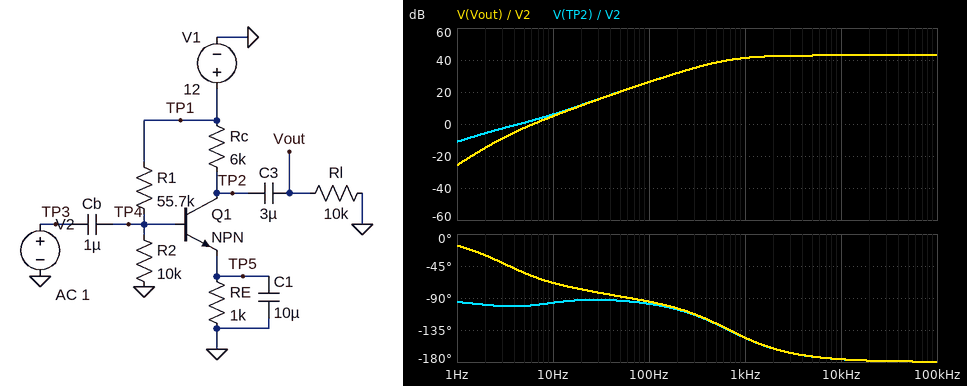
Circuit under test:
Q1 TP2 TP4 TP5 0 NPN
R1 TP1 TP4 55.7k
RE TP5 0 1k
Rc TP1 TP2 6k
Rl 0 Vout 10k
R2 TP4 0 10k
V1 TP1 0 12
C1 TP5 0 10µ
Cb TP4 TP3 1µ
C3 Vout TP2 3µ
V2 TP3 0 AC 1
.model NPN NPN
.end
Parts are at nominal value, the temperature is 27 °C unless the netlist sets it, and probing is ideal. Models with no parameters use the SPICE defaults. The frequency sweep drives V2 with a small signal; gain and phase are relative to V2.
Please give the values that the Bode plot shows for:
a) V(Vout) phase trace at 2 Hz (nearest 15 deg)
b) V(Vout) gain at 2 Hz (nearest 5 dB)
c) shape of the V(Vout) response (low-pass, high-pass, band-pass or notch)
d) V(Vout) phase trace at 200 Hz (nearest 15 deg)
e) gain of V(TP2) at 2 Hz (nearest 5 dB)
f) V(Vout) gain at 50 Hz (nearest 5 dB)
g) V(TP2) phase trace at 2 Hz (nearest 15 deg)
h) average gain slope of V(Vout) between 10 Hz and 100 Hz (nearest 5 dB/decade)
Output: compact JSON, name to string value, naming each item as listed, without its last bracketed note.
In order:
{"V(Vout) phase trace at 2 Hz": "-30 deg", "V(Vout) gain at 2 Hz": "-15 dB", "shape of the V(Vout) response": "high-pass", "V(Vout) phase trace at 200 Hz": "-105 deg", "gain of V(TP2) at 2 Hz": "-5 dB", "V(Vout) gain at 50 Hz": "20 dB", "V(TP2) phase trace at 2 Hz": "-105 deg", "average gain slope of V(Vout) between 10 Hz and 100 Hz": "20 dB/decade"}
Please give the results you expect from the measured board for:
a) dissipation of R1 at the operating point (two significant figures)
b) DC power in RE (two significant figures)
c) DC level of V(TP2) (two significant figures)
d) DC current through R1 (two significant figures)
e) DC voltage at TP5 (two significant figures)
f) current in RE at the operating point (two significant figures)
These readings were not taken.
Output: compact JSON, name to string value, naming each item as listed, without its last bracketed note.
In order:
{"dissipation of R1 at the operating point": "1.9 mW", "DC power in RE": "940 µW", "DC level of V(TP2)": "6.2 V", "DC current through R1": "180 µA", "DC voltage at TP5": "970 mV", "current in RE at the operating point": "970 µA"}
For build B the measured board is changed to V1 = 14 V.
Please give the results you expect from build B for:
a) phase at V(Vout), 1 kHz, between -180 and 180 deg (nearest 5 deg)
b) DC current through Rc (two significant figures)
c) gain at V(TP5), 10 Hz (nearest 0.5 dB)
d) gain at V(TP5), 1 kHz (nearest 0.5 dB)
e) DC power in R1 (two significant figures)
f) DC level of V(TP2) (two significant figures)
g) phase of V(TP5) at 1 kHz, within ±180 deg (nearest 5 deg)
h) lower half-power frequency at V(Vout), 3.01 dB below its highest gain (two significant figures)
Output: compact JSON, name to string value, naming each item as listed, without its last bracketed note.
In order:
{"phase at V(Vout), 1 kHz, between -180 and 180 deg": "-140 deg", "DC current through Rc": "1.2 mA", "gain at V(TP5), 10 Hz": "-7.5 dB", "gain at V(TP5), 1 kHz": "-4.5 dB", "DC power in R1": "2.6 mW", "DC level of V(TP2)": "6.6 V", "phase of V(TP5) at 1 kHz, within ±180 deg": "-50 deg", "lower half-power frequency at V(Vout), 3.01 dB below its highest gain": "860 Hz"}
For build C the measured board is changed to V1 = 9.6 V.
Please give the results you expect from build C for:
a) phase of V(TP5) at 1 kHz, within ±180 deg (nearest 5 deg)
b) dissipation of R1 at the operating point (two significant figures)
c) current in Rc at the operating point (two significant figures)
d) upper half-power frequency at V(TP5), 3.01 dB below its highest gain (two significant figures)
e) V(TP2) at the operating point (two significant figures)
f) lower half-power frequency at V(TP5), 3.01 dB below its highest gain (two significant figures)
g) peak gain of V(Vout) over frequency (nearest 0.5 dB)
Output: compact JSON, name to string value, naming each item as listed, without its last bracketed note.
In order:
{"phase of V(TP5) at 1 kHz, within ±180 deg": "-65 deg", "dissipation of R1 at the operating point": "1.2 mW", "current in Rc at the operating point": "640 µA", "upper half-power frequency at V(TP5), 3.01 dB below its highest gain": "490 Hz", "V(TP2) at the operating point": "5.8 V", "lower half-power frequency at V(TP5), 3.01 dB below its highest gain": "17 Hz", "peak gain of V(Vout) over frequency": "39.5 dB"}
